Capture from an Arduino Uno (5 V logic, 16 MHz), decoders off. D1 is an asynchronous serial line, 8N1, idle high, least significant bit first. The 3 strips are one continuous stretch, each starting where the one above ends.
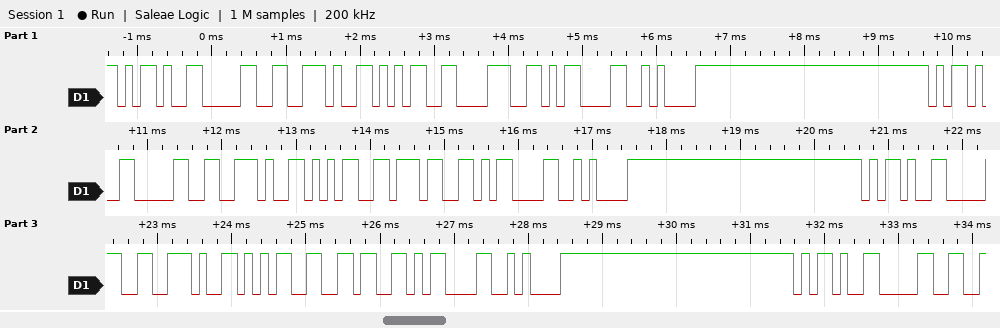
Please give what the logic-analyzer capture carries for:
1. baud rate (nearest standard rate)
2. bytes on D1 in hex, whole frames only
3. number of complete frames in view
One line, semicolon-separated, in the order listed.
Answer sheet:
9600 baud; 2D 30 2E 35 38 0D 0A 2D 30 2E 35 37 0D 0A 2D 30 2E 35 36 0D 0A 2D 30; 23
